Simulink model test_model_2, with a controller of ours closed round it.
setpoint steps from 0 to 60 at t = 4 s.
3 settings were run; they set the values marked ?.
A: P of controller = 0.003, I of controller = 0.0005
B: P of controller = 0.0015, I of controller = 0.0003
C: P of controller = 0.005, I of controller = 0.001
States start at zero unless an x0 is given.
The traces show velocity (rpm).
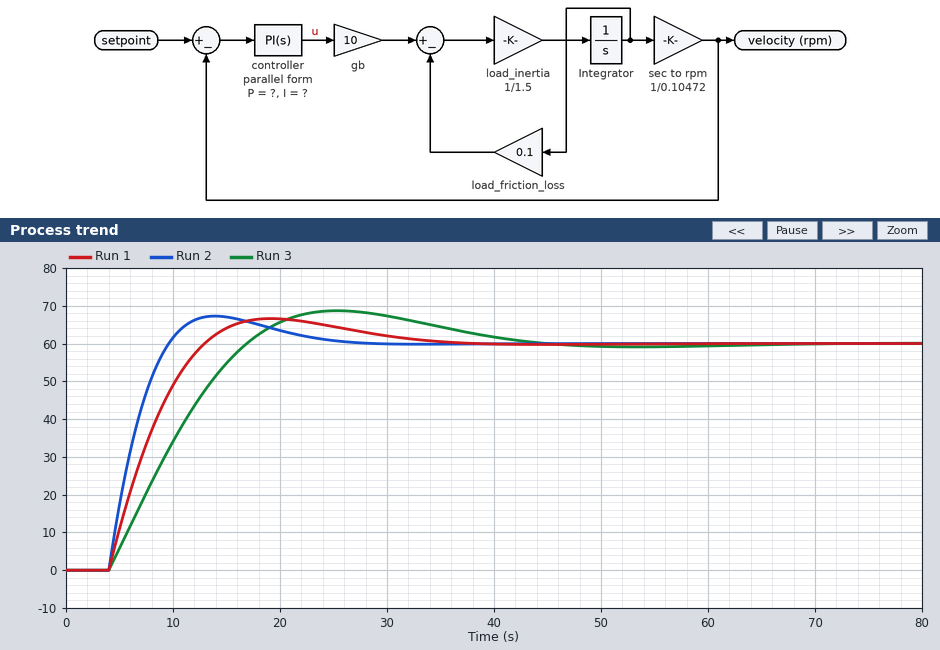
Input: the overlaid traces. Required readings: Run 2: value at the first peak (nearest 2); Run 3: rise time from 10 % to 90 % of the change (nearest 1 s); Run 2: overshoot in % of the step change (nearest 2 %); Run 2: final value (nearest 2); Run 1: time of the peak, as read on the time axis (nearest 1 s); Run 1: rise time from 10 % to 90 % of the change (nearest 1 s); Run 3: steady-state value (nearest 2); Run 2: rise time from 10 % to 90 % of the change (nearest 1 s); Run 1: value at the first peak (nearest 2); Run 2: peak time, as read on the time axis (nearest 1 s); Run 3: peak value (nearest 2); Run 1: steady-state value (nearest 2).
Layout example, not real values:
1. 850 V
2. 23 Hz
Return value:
1. 68
2. 10 s
3. 12 %
4. 60
5. 19 s
6. 7 s
7. 60
8. 4 s
9. 66
10. 14 s
11. 68
12. 60
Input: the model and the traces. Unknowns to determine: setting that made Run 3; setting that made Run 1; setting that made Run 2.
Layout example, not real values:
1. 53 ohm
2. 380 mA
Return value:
1. B
2. A
3. C
